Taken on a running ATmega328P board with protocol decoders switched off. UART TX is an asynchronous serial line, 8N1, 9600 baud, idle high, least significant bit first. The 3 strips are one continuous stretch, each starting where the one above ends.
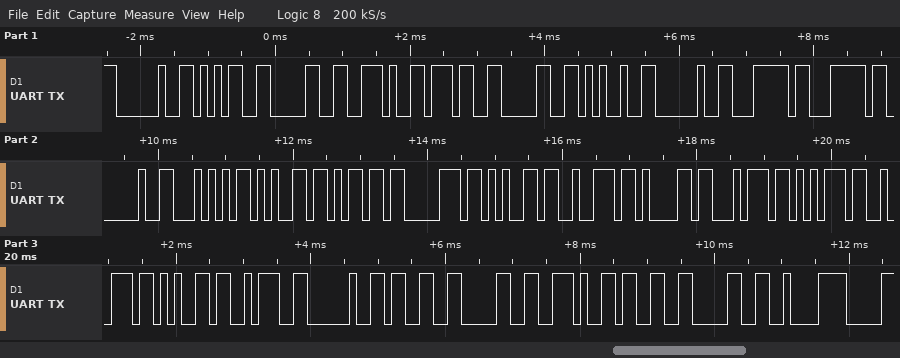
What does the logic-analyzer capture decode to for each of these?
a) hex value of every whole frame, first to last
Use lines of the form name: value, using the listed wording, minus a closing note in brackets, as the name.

hex value of every whole frame, first to last: 20 35 30 2E 37 30 25 20 7C 7C 20 54 65 6D 70 65 72 61 74 75 72 65 3A 20 33 30 2E 33 30 C2
